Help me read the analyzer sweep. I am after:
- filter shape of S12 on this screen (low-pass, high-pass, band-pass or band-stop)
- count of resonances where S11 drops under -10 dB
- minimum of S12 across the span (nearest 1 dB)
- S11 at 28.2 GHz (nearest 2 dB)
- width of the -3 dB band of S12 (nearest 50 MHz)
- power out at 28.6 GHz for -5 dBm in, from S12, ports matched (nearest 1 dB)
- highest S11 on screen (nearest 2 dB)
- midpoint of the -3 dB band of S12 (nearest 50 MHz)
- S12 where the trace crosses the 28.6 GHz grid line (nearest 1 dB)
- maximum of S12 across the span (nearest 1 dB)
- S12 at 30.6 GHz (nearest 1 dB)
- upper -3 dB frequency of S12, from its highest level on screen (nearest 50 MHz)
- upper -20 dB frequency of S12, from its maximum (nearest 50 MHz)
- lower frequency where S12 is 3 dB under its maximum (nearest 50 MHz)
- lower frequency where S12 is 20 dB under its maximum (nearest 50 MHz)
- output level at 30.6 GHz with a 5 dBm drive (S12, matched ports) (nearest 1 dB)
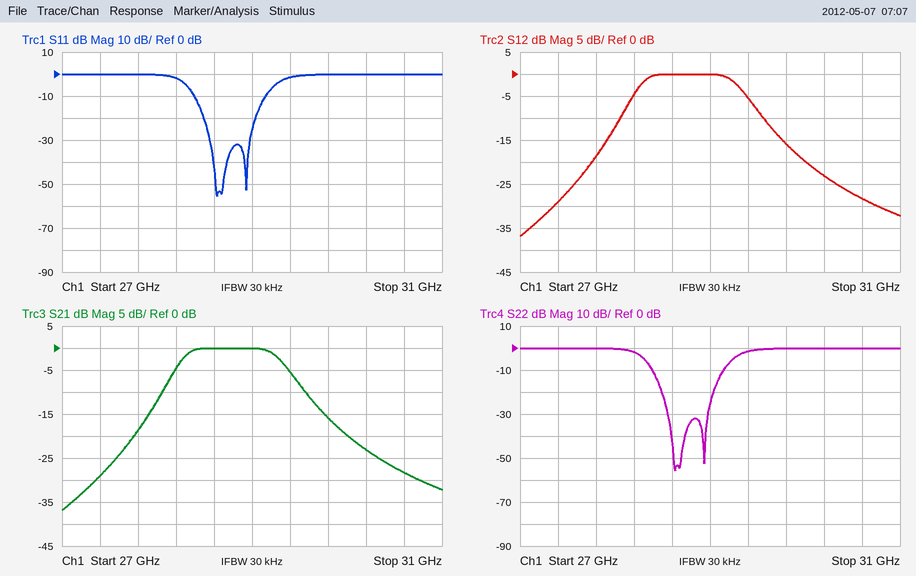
band-pass
2
-37 dB
-2 dB
1.05 GHz
-5 dBm
0 dB
28.80 GHz
0 dB
0 dB
-28 dB
29.30 GHz
30.00 GHz
28.25 GHz
27.75 GHz
-23 dBm
